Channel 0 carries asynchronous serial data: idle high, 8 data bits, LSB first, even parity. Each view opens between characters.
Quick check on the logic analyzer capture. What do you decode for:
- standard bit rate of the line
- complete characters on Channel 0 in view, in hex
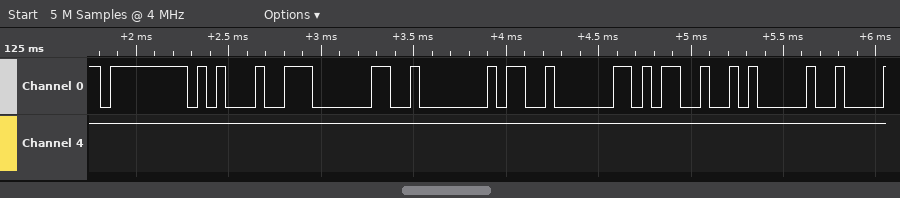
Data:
19200 baud
FF, 91, 60, 40, 02, 4D, 41
